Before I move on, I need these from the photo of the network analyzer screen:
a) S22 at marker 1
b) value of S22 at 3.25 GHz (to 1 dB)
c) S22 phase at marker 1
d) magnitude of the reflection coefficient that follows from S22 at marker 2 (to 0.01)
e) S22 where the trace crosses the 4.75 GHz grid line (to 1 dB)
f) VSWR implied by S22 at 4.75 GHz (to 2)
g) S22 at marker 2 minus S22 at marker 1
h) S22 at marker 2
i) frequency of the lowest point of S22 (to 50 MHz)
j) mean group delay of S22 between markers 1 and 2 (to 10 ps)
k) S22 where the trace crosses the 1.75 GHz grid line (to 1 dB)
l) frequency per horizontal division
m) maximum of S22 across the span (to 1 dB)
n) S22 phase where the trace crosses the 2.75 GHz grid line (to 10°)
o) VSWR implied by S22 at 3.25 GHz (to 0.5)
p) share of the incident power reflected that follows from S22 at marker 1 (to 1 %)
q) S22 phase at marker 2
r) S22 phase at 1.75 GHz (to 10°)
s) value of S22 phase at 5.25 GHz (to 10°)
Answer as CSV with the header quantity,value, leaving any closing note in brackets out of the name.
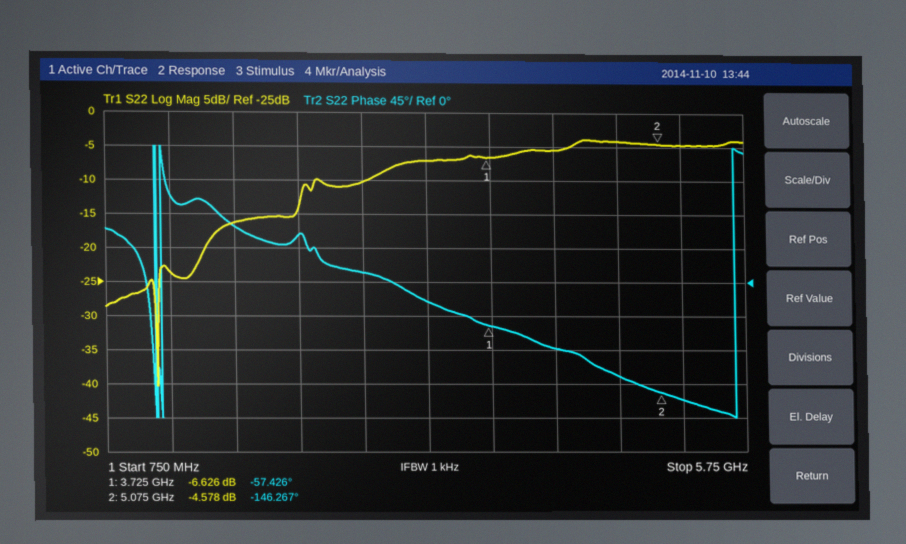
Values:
quantity,value
S22 at marker 1,-6.626 dB
value of S22 at 3.25 GHz,-7 dB
S22 phase at marker 1,-57.426°
magnitude of the reflection coefficient that follows from S22 at marker 2,0.59
S22 where the trace crosses the 4.75 GHz grid line,-4 dB
VSWR implied by S22 at 4.75 GHz,4
S22 at marker 2 minus S22 at marker 1,2.048 dB
S22 at marker 2,-4.578 dB
frequency of the lowest point of S22,1.15 GHz
mean group delay of S22 between markers 1 and 2,180 ps
S22 where the trace crosses the 1.75 GHz grid line,-16 dB
frequency per horizontal division,500 MHz
maximum of S22 across the span,-4 dB
S22 phase where the trace crosses the 2.75 GHz grid line,10°
VSWR implied by S22 at 3.25 GHz,2.5
share of the incident power reflected that follows from S22 at marker 1,22 %
S22 phase at marker 2,-146.267°
S22 phase at 1.75 GHz,70°
value of S22 phase at 5.25 GHz,-160°
